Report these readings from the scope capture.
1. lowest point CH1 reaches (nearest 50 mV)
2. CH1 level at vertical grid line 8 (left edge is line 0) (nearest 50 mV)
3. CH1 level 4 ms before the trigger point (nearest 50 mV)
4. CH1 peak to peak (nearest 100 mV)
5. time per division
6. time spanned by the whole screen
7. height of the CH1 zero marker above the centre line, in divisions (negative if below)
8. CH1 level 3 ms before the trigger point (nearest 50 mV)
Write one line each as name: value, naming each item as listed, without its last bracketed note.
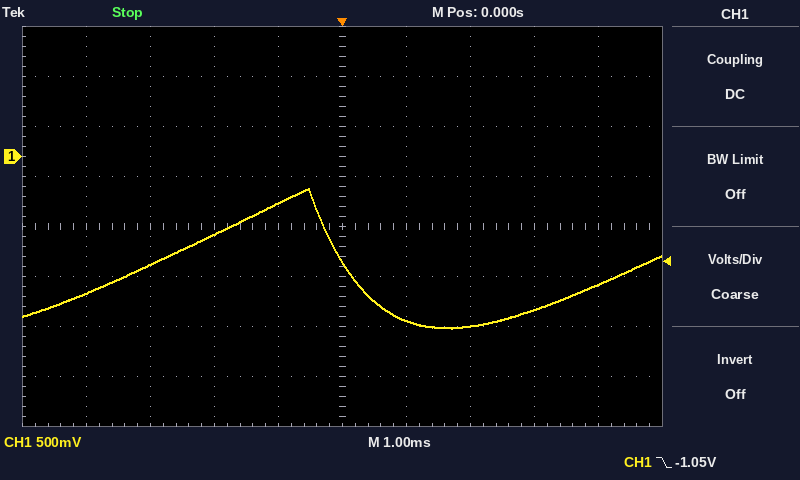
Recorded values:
lowest point CH1 reaches: -1.70 V
CH1 level at vertical grid line 8 (left edge is line 0): -1.55 V
CH1 level 4 ms before the trigger point: -1.35 V
CH1 peak to peak: 1.40 V
time per division: 1 ms
time spanned by the whole screen: 10 ms
height of the CH1 zero marker above the centre line, in divisions: +1.4 div
CH1 level 3 ms before the trigger point: -1.10 V
